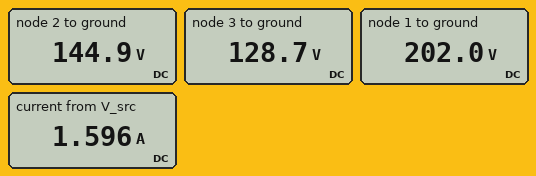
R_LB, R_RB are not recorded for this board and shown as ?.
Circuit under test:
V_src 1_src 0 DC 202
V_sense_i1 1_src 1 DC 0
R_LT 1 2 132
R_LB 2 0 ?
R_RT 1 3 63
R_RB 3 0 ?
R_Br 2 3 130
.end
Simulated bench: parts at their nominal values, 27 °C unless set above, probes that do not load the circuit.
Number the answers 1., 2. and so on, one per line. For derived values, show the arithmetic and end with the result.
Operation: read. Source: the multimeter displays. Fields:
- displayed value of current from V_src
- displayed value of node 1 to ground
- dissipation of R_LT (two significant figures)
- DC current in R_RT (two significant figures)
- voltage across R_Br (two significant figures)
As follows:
1. 1.596 A
2. 202.0 V
3. (202 V - 144.9 V)^2 / 132 Ω = 25 W
4. (202 V - 128.7 V) / 63 Ω = 1.2 A
5. 144.9 V - 128.7 V = 16 V
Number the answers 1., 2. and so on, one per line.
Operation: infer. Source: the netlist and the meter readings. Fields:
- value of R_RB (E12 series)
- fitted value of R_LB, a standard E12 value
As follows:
1. 100 Ω
2. 470 Ω
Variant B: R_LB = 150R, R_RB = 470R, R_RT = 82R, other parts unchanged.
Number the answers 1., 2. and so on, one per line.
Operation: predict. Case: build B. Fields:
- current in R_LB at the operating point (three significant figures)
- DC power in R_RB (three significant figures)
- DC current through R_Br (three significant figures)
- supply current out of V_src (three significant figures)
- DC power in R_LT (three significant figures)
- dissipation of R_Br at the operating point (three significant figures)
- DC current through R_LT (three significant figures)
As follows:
1. 828 mA
2. 51.3 W
3. 239 mA
4. 1.16 A
5. 45.8 W
6. 7.43 W
7. 589 mA
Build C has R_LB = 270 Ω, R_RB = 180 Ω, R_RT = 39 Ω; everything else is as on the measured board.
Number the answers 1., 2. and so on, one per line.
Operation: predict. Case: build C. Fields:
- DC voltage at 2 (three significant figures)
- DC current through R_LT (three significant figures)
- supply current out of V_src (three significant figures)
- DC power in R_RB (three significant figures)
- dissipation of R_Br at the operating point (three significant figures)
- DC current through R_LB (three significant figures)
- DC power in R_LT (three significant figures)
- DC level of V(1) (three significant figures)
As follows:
1. 146 V
2. 421 mA
3. 1.44 A
4. 146 W
5. 1.91 W
6. 542 mA
7. 23.4 W
8. 202 V
